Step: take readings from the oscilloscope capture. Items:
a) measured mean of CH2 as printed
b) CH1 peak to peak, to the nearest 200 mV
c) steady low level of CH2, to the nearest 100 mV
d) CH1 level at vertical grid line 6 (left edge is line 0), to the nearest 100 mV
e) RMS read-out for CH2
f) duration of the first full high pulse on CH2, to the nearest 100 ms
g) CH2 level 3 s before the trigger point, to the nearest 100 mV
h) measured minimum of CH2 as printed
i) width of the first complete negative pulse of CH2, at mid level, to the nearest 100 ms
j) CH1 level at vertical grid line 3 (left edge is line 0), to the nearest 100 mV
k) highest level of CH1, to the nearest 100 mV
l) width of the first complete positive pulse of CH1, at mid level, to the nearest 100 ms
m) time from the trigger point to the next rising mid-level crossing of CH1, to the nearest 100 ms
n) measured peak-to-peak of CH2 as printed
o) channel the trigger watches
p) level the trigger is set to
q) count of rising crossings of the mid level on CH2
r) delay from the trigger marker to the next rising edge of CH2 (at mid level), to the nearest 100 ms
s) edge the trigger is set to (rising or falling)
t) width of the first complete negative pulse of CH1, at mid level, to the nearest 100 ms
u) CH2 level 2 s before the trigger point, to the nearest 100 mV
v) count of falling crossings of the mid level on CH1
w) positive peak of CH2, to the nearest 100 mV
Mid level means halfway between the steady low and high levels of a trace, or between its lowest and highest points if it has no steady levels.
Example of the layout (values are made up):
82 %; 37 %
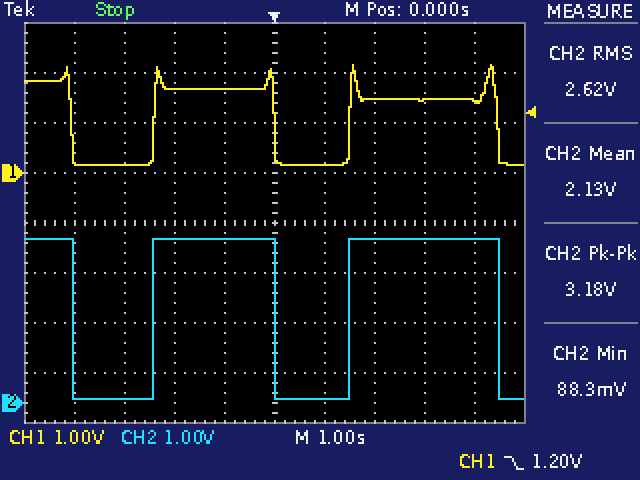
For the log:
2.13 V; 2.0 V; 100 mV; 200 mV; 2.62 V; 2.4 s; 100 mV; 88.3 mV; 1.6 s; 1.7 V; 2.2 V; 2.4 s; 1.5 s; 3.18 V; CH1; 1.20 V; 2; 1.5 s; falling; 1.7 s; 3.3 V; 3; 3.3 V
